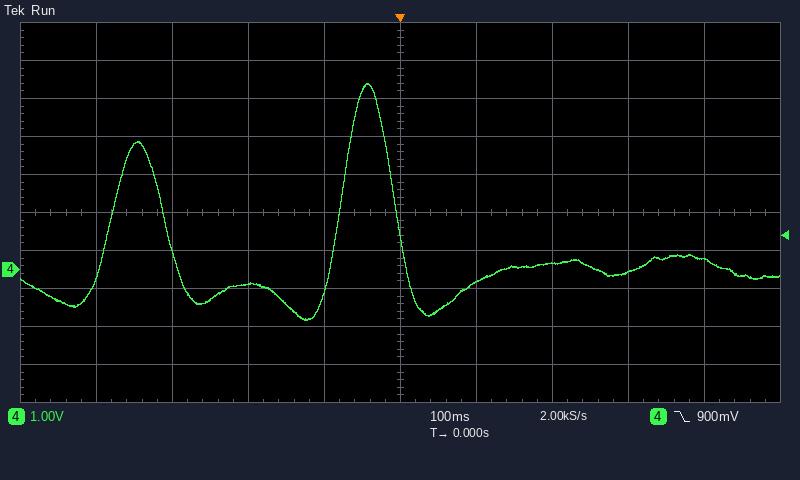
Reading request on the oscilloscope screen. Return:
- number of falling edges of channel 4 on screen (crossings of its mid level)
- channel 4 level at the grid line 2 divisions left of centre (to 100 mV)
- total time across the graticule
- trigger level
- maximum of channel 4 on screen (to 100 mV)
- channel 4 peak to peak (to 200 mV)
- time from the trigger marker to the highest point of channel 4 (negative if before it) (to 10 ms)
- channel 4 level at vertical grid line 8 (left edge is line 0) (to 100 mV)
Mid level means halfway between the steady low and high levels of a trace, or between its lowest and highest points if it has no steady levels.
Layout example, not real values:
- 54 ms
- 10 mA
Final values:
- 2
- -400 mV
- 1 s
- 900 mV
- 4.9 V
- 6.2 V
- -40 ms
- -100 mV
